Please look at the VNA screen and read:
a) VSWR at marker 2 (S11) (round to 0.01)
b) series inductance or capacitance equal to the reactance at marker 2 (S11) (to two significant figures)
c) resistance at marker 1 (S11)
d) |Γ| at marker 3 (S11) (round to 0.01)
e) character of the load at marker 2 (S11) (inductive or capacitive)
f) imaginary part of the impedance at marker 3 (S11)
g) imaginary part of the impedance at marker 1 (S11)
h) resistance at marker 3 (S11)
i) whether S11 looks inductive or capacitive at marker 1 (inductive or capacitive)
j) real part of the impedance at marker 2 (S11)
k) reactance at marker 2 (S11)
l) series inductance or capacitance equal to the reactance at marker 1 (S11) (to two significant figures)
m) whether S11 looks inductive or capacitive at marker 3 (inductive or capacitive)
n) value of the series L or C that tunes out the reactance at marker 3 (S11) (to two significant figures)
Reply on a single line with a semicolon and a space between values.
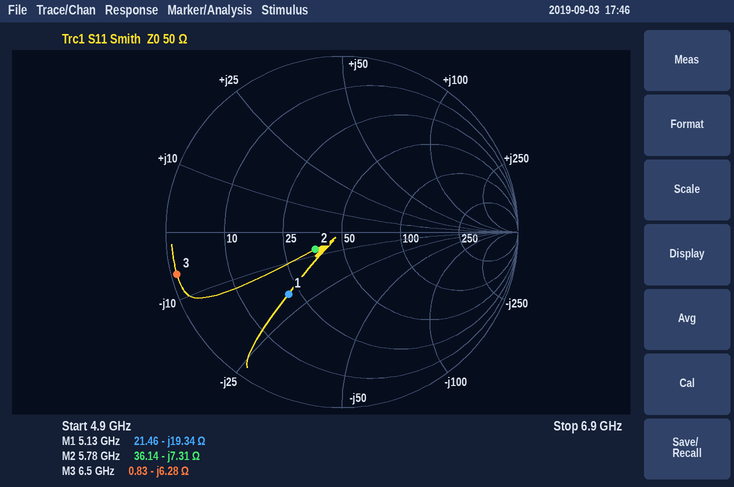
1.44; 3.8 pF; 21.46 Ω; 0.97; capacitive; -6.28 Ω; -19.34 Ω; 0.83 Ω; capacitive; 36.14 Ω; -7.31 Ω; 1.6 pF; capacitive; 150 pH
